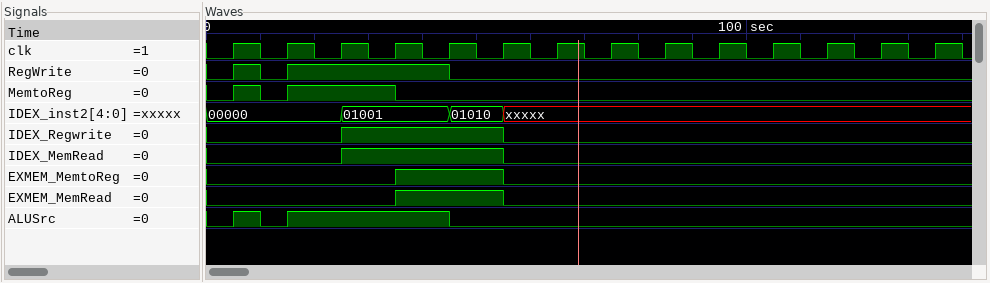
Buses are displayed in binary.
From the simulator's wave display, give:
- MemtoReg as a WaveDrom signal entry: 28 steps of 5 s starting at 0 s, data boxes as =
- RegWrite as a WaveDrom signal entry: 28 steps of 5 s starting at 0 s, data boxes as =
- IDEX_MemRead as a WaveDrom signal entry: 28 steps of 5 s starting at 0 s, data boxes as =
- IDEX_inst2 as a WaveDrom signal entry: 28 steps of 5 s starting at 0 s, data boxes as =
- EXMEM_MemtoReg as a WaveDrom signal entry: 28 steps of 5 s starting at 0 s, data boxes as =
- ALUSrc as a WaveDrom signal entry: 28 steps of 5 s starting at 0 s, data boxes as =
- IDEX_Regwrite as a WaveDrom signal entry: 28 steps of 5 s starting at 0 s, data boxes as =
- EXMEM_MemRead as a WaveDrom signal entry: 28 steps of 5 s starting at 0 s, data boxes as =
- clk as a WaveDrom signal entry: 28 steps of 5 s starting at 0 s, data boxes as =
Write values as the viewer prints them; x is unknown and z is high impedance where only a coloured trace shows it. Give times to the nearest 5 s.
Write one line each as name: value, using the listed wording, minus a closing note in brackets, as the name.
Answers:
MemtoReg as a WaveDrom signal entry: 28 steps of 5 s starting at 0 s, data boxes as =: {name: 'MemtoReg', wave: '0101...0....................'}
RegWrite as a WaveDrom signal entry: 28 steps of 5 s starting at 0 s, data boxes as =: {name: 'RegWrite', wave: '0101.....0..................'}
IDEX_MemRead as a WaveDrom signal entry: 28 steps of 5 s starting at 0 s, data boxes as =: {name: 'IDEX_MemRead', wave: '0....1.....0................'}
IDEX_inst2 as a WaveDrom signal entry: 28 steps of 5 s starting at 0 s, data boxes as =: {name: 'IDEX_inst2', wave: '=....=...=.x................', data: '00000 01001 01010'}
EXMEM_MemtoReg as a WaveDrom signal entry: 28 steps of 5 s starting at 0 s, data boxes as =: {name: 'EXMEM_MemtoReg', wave: '0......1...0................'}
ALUSrc as a WaveDrom signal entry: 28 steps of 5 s starting at 0 s, data boxes as =: {name: 'ALUSrc', wave: '0101.....0..................'}
IDEX_Regwrite as a WaveDrom signal entry: 28 steps of 5 s starting at 0 s, data boxes as =: {name: 'IDEX_Regwrite', wave: '0....1.....0................'}
EXMEM_MemRead as a WaveDrom signal entry: 28 steps of 5 s starting at 0 s, data boxes as =: {name: 'EXMEM_MemRead', wave: '0......1...0................'}
clk as a WaveDrom signal entry: 28 steps of 5 s starting at 0 s, data boxes as =: {name: 'clk', wave: '0101010101010101010101010101'}
